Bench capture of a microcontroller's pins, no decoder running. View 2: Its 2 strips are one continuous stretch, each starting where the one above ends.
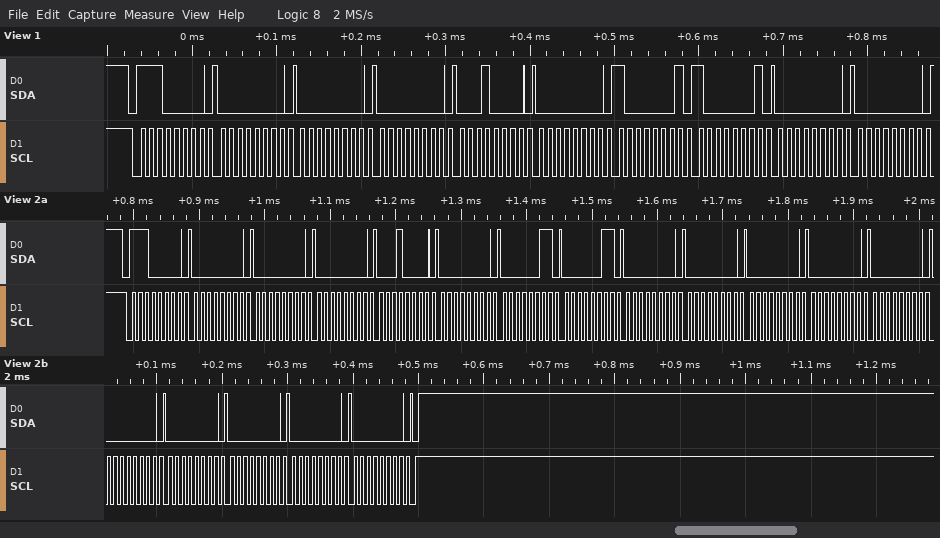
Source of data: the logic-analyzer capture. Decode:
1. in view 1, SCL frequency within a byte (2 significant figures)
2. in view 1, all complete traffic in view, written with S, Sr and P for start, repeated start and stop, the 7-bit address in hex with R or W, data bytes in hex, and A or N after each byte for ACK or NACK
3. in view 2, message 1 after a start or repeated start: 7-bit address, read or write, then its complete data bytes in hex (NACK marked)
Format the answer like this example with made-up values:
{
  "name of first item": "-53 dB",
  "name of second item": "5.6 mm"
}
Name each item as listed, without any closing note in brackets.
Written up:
{
  "in view 1, SCL frequency within a byte": "100 kHz",
  "in view 1, all complete traffic in view, written with S, Sr and P for start, repeated start and stop, the 7-bit address in hex with R or W, data bytes in hex, and A or N after each byte for ACK or NACK": "S 70W A 00 A 00 A 00 A 10 A 00 A 81 A 81 A 00 A 00 A",
  "in view 2, message 1 after a start or repeated start: 7-bit address, read or write, then its complete data bytes in hex": "0x70 write: 00 00 00 10 00 03 03 00 00 00 00 00 00 00 00 00 00"
}
